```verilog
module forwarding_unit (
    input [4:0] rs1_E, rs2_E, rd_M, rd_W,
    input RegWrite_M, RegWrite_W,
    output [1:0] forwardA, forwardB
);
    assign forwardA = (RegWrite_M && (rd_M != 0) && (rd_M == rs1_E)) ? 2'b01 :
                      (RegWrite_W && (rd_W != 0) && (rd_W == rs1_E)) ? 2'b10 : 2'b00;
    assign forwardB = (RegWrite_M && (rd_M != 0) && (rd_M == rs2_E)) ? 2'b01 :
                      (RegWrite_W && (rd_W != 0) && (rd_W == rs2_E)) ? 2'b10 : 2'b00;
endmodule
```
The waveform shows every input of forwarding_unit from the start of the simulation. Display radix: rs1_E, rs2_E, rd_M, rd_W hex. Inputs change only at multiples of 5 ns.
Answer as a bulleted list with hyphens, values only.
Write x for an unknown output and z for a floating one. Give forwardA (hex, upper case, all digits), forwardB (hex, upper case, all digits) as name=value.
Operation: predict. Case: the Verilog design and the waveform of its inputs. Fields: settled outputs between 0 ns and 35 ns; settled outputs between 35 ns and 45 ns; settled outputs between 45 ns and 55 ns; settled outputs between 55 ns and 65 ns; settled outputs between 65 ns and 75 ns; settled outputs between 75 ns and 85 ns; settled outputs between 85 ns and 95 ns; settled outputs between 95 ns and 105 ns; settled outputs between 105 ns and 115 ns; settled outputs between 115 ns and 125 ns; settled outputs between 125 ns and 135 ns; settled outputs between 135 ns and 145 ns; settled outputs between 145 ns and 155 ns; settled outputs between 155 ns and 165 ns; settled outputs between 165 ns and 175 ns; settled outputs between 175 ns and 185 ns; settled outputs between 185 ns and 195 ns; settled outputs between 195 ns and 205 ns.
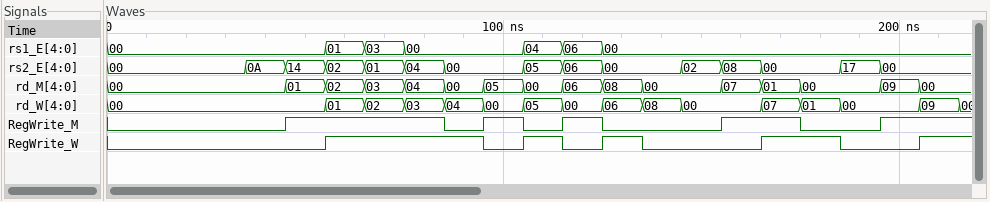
- forwardA=0, forwardB=0
- forwardA=0, forwardB=0
- forwardA=0, forwardB=0
- forwardA=2, forwardB=1
- forwardA=1, forwardB=0
- forwardA=0, forwardB=1
- forwardA=0, forwardB=0
- forwardA=0, forwardB=0
- forwardA=0, forwardB=2
- forwardA=1, forwardB=1
- forwardA=0, forwardB=0
- forwardA=0, forwardB=0
- forwardA=0, forwardB=0
- forwardA=0, forwardB=0
- forwardA=0, forwardB=0
- forwardA=0, forwardB=0
- forwardA=0, forwardB=0
- forwardA=0, forwardB=0
